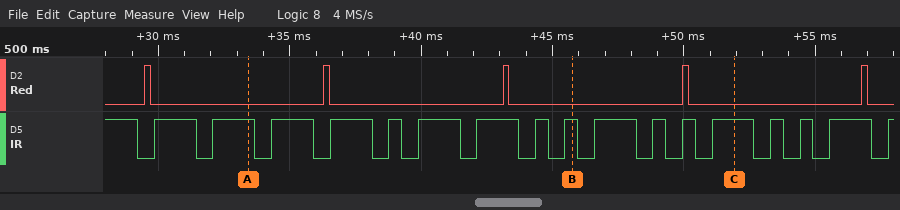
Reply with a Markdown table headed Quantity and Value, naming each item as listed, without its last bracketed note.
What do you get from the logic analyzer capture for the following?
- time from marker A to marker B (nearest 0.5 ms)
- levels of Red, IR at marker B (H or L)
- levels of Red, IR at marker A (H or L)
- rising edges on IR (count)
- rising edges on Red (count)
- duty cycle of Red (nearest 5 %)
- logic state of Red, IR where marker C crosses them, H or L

| Quantity | Value |
|---|---|
| time from marker A to marker B | 12.5 ms |
| levels of Red, IR at marker B | Red=L, IR=H |
| levels of Red, IR at marker A | Red=L, IR=H |
| rising edges on IR | 17 |
| rising edges on Red | 5 |
| duty cycle of Red | 5 % |
| logic state of Red, IR where marker C crosses them, H or L | Red=L, IR=H |
